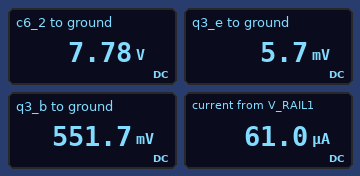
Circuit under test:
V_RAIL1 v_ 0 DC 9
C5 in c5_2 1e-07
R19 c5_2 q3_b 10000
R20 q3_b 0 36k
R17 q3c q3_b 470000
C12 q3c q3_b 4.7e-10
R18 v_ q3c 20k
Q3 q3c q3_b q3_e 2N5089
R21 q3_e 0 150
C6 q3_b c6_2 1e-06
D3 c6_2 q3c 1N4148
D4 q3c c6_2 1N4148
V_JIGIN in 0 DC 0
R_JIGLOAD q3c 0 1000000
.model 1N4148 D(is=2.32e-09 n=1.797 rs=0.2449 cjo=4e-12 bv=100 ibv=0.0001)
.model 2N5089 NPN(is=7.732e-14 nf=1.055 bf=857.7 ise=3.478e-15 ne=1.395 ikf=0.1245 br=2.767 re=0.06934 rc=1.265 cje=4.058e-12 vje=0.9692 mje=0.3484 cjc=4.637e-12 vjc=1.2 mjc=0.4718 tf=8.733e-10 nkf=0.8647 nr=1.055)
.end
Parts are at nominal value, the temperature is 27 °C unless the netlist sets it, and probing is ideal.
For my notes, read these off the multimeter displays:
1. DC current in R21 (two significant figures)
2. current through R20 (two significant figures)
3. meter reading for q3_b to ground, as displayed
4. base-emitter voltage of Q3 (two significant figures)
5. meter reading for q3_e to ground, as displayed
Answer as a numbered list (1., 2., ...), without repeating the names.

1. 38 µA
2. 15 µA
3. 551.7 mV
4. 550 mV
5. 5.7 mV
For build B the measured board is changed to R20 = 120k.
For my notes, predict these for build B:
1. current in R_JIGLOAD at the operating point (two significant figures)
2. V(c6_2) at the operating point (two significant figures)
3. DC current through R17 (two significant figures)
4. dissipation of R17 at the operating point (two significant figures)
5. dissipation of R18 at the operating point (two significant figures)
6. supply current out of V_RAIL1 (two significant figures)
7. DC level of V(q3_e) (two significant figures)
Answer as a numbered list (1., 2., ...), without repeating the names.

1. 3.3 µA
2. 3.3 V
3. 5.7 µA
4. 15 µW
5. 1.6 mW
6. 280 µA
7. 41 mV
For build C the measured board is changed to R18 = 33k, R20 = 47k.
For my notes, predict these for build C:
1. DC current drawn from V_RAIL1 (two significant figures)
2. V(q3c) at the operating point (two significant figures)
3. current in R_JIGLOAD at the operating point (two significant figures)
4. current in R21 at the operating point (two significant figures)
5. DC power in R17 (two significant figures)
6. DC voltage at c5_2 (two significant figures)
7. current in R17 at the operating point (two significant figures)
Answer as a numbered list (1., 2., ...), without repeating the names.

1. 82 µA
2. 6.3 V
3. 6.3 µA
4. 63 µA
5. 70 µW
6. 570 mV
7. 12 µA
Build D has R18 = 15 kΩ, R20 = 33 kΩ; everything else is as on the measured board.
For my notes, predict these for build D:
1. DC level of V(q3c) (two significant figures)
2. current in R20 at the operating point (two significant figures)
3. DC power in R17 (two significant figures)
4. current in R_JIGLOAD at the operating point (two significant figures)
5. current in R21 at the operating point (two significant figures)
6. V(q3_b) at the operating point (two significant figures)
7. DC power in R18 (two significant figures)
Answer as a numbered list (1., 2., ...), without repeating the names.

1. 8.2 V
2. 16 µA
3. 130 µW
4. 8.2 µA
5. 26 µA
6. 540 mV
7. 38 µW
